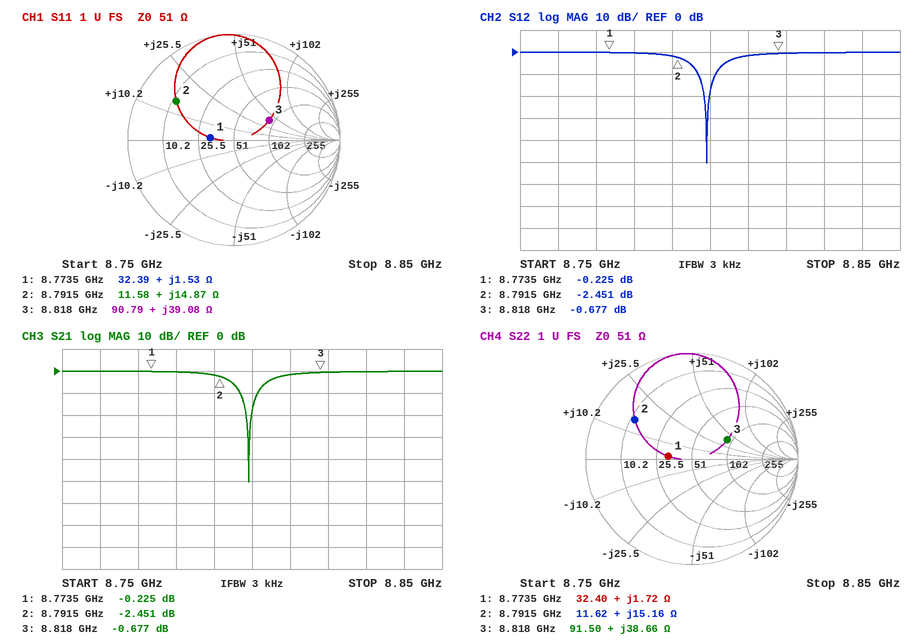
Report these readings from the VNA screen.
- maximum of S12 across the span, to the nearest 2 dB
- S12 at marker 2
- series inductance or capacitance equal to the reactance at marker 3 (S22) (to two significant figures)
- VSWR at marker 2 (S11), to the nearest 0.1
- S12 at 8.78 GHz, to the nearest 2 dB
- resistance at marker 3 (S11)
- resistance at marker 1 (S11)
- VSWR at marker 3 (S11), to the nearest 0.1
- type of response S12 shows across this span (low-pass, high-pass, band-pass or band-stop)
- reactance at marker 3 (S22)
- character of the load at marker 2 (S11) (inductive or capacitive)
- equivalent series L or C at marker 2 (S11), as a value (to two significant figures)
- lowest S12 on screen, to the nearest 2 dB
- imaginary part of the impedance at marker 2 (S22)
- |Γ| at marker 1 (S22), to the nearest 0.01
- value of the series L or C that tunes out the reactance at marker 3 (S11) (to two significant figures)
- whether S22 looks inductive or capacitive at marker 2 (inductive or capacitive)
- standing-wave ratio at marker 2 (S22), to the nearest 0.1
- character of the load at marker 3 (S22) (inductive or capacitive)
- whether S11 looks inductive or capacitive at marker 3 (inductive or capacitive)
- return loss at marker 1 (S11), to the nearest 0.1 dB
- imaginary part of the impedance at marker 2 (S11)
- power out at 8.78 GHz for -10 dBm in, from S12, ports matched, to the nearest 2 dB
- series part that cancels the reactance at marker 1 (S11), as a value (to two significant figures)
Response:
0 dB
-2.451 dB
700 pH
4.8
0 dB
90.79 Ω
32.39 Ω
2.2
band-stop
+38.66 Ω
inductive
270 pH
-50 dB
+15.16 Ω
0.22
460 fF
inductive
4.8
inductive
inductive
13.0 dB
+14.87 Ω
-10 dBm
12 pF
